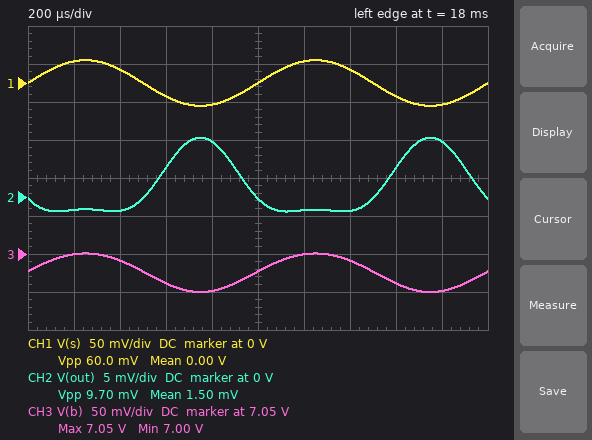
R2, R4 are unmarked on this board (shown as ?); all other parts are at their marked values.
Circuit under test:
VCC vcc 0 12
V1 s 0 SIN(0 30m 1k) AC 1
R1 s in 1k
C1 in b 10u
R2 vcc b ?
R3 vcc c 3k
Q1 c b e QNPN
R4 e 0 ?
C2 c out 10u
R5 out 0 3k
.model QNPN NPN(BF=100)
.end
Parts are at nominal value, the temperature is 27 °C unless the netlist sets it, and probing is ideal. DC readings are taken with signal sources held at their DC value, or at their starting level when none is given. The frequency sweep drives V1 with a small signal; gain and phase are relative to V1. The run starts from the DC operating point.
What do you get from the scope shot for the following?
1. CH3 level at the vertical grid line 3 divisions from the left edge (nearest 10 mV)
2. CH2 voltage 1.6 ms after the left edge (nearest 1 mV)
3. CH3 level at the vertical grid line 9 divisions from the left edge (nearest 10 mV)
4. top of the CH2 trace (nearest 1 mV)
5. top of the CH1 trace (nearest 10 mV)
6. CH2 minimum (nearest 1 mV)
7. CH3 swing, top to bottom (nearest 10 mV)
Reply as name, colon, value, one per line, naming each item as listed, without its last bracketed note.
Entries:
CH3 level at the vertical grid line 3 divisions from the left edge: 7.01 V
CH2 voltage 1.6 ms after the left edge: 4 mV
CH3 level at the vertical grid line 9 divisions from the left edge: 7.00 V
top of the CH2 trace: 8 mV
top of the CH1 trace: 30 mV
CH2 minimum: -2 mV
CH3 swing, top to bottom: 50 mV
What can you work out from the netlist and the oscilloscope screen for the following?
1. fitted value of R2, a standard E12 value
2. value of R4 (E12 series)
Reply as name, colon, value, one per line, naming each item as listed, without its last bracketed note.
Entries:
fitted value of R2, a standard E12 value: 220 kΩ
value of R4: 3.3 kΩ
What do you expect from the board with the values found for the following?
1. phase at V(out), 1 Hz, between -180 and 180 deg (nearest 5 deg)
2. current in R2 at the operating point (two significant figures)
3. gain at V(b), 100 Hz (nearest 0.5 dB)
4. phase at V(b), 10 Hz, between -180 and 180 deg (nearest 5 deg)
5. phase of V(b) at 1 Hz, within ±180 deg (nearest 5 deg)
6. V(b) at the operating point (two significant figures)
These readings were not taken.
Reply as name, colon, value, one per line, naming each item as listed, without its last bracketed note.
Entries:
phase at V(out), 1 Hz, between -180 and 180 deg: -35 deg
current in R2 at the operating point: 23 µA
gain at V(b), 100 Hz: -1.5 dB
phase at V(b), 10 Hz, between -180 and 180 deg: 15 deg
phase of V(b) at 1 Hz, within ±180 deg: 70 deg
V(b) at the operating point: 7.0 V
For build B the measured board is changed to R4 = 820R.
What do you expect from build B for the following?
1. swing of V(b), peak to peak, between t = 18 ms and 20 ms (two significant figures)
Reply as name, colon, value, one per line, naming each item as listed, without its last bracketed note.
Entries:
swing of V(b), peak to peak, between t = 18 ms and 20 ms: 40 mV
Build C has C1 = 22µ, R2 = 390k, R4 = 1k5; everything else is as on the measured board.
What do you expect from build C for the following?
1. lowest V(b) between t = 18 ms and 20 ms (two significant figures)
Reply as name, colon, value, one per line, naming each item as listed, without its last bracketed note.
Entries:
lowest V(b) between t = 18 ms and 20 ms: 3.9 V
